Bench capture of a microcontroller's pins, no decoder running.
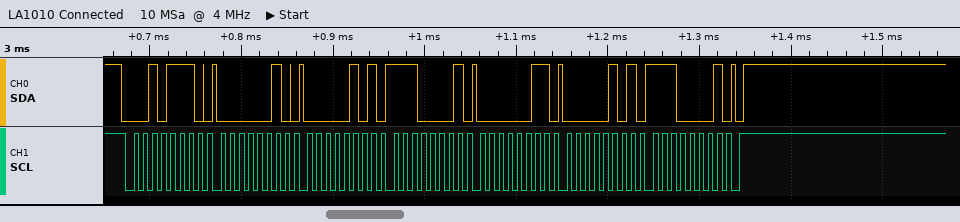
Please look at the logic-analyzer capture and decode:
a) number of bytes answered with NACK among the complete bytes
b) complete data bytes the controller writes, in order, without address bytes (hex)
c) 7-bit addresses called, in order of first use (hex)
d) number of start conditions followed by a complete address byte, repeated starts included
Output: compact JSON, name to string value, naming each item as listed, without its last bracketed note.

{"number of bytes answered with NACK among the complete bytes": "0", "complete data bytes the controller writes, in order, without address bytes": "02 05 E1 03 05 E1", "7-bit addresses called, in order of first use": "0x17", "number of start conditions followed by a complete address byte, repeated starts included": "1"}
